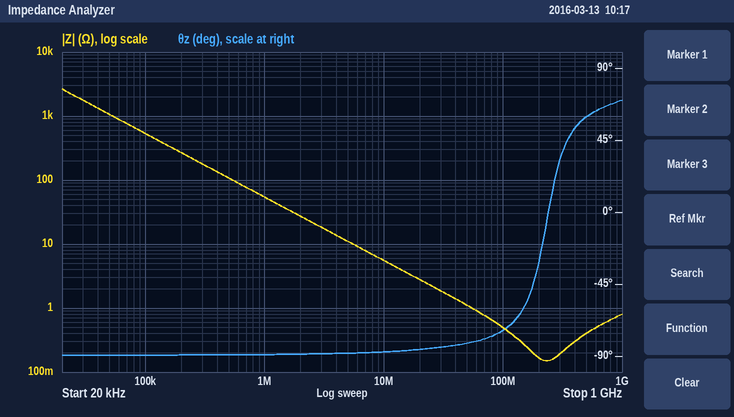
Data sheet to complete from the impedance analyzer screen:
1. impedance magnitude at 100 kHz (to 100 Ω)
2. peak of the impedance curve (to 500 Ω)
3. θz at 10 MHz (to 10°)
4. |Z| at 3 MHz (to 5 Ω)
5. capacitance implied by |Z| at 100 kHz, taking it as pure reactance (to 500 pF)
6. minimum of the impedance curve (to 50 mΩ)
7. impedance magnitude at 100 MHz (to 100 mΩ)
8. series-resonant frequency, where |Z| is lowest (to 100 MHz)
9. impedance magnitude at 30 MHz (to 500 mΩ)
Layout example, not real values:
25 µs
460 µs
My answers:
500 Ω
2.5 kΩ
-90°
20 Ω
3.0 nF
150 mΩ
500 mΩ
200 MHz
2.0 Ω
